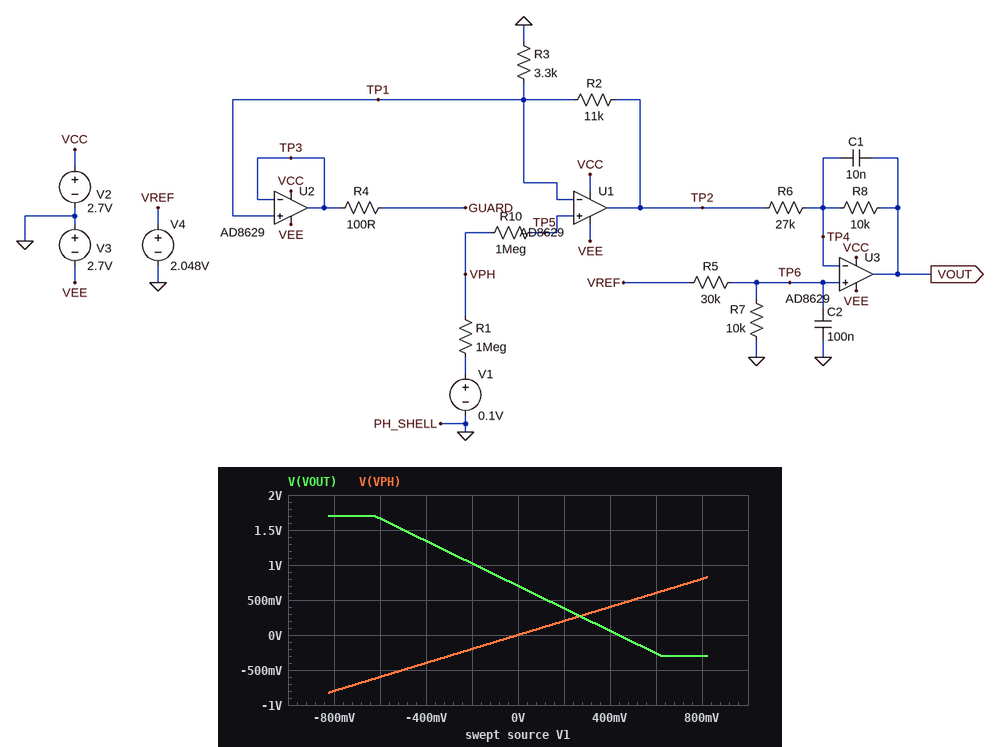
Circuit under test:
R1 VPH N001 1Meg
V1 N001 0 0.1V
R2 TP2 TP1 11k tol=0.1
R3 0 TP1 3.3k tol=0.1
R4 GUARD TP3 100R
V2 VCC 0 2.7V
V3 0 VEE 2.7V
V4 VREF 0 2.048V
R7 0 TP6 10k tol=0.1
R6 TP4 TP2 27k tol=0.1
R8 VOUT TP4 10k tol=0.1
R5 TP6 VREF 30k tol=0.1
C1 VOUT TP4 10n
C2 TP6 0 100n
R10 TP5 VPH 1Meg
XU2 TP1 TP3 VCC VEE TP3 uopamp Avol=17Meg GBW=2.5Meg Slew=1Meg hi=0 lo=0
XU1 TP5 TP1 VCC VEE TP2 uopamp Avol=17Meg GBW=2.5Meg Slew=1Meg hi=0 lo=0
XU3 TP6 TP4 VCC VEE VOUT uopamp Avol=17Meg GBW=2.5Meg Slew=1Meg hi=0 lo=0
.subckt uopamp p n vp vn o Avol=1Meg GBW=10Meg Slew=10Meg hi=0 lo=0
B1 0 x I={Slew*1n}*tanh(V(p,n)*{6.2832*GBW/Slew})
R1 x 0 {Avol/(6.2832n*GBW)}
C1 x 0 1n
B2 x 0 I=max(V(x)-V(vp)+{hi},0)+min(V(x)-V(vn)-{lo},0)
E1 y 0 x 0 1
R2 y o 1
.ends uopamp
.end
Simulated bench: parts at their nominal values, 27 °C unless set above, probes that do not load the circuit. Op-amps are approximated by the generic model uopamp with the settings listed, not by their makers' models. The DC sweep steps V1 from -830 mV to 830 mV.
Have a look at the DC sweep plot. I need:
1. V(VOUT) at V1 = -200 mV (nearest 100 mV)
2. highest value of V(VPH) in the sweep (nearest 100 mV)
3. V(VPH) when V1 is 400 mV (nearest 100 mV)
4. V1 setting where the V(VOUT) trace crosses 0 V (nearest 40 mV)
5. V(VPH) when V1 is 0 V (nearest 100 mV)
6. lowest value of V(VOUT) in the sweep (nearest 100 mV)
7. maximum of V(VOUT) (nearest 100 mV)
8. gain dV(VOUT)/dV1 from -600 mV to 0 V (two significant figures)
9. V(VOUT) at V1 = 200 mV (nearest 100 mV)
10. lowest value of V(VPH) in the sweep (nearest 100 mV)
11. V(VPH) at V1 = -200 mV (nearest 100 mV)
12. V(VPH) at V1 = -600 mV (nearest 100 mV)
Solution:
1.0 V
800 mV
400 mV
440 mV
0 V
-300 mV
1.7 V
-1.6 V/V
400 mV
-800 mV
-200 mV
-600 mV
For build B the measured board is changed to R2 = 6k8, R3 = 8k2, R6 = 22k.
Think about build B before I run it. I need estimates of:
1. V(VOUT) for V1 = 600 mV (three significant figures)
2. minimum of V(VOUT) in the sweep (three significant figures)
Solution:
246 mV
54.6 mV
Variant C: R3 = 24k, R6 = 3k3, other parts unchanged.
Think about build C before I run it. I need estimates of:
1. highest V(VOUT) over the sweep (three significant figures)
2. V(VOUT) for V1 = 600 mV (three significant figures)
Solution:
2.70 V
-588 mV
